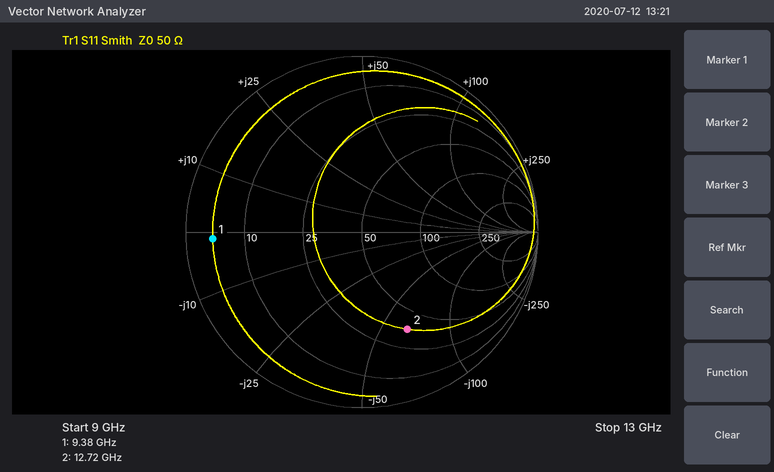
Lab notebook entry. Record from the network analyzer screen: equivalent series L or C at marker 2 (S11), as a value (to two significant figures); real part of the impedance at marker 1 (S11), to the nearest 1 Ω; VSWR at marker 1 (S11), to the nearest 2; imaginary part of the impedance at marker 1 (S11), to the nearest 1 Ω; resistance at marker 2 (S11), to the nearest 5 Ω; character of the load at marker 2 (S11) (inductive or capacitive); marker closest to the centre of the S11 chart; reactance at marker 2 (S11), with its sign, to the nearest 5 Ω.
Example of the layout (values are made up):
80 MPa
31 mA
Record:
190 fF
4 Ω
12
-1 Ω
35 Ω
capacitive
marker 2
-65 Ω
